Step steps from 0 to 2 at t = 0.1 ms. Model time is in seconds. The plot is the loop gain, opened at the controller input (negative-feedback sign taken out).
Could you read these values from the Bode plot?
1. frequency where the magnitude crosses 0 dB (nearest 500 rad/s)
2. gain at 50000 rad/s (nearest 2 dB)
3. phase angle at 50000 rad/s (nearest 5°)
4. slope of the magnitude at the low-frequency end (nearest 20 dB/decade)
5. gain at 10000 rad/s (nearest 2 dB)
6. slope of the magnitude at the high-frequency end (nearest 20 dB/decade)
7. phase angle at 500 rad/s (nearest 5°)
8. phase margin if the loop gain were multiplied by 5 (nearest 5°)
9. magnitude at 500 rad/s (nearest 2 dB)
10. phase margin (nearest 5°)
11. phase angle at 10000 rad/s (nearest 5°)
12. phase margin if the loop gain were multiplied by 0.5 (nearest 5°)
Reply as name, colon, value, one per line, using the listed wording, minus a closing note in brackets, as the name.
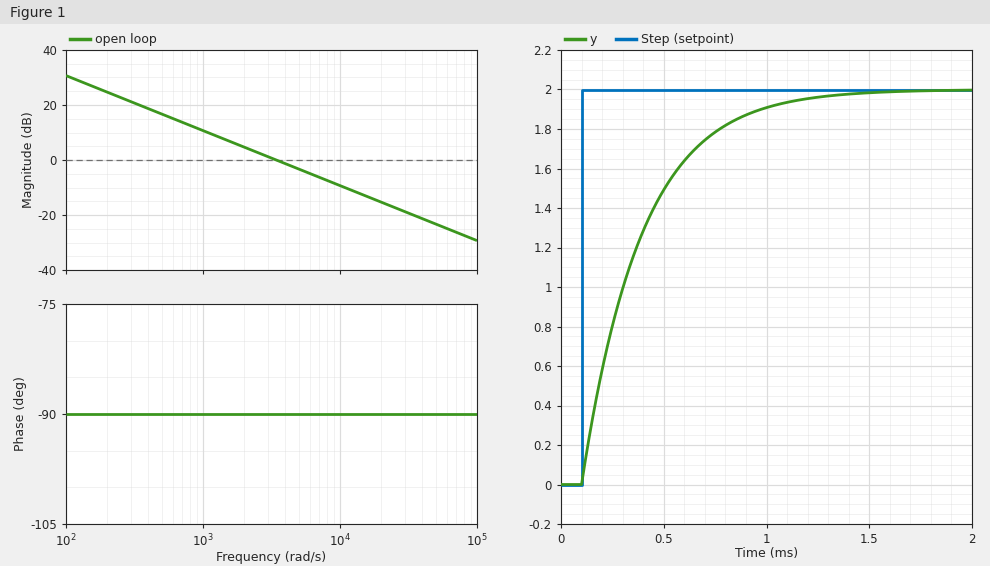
frequency where the magnitude crosses 0 dB: 3500 rad/s
gain at 50000 rad/s: -24 dB
phase angle at 50000 rad/s: -90°
slope of the magnitude at the low-frequency end: -20 dB/decade
gain at 10000 rad/s: -10 dB
slope of the magnitude at the high-frequency end: -20 dB/decade
phase angle at 500 rad/s: -90°
phase margin if the loop gain were multiplied by 5: 90°
magnitude at 500 rad/s: 16 dB
phase margin: 90°
phase angle at 10000 rad/s: -90°
phase margin if the loop gain were multiplied by 0.5: 90°
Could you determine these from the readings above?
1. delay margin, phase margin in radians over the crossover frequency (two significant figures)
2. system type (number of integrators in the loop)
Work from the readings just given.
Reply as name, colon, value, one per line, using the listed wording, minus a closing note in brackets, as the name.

delay margin, phase margin in radians over the crossover frequency: 0.00045 s
system type: 1
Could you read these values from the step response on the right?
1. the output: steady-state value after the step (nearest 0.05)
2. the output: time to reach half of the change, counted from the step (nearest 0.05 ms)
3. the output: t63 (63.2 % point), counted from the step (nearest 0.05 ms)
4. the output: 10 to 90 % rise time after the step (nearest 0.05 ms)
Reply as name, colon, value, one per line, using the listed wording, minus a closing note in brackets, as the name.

the output: steady-state value after the step: 2.00
the output: time to reach half of the change, counted from the step: 0.20 ms
the output: t63 (63.2 % point), counted from the step: 0.30 ms
the output: 10 to 90 % rise time after the step: 0.65 ms
